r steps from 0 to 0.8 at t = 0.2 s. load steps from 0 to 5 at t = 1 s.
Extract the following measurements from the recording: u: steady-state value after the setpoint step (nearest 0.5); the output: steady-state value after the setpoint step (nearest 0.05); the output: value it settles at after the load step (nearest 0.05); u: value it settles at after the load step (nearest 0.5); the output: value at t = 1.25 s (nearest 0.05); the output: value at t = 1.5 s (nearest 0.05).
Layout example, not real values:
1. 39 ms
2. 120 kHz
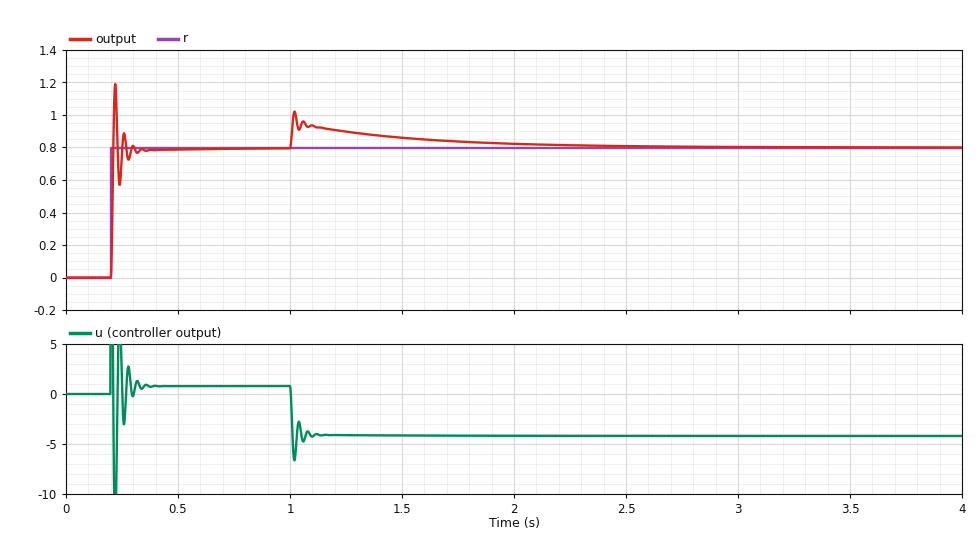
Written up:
1. 1.0
2. 0.80
3. 0.80
4. -4.0
5. 0.90
6. 0.85
